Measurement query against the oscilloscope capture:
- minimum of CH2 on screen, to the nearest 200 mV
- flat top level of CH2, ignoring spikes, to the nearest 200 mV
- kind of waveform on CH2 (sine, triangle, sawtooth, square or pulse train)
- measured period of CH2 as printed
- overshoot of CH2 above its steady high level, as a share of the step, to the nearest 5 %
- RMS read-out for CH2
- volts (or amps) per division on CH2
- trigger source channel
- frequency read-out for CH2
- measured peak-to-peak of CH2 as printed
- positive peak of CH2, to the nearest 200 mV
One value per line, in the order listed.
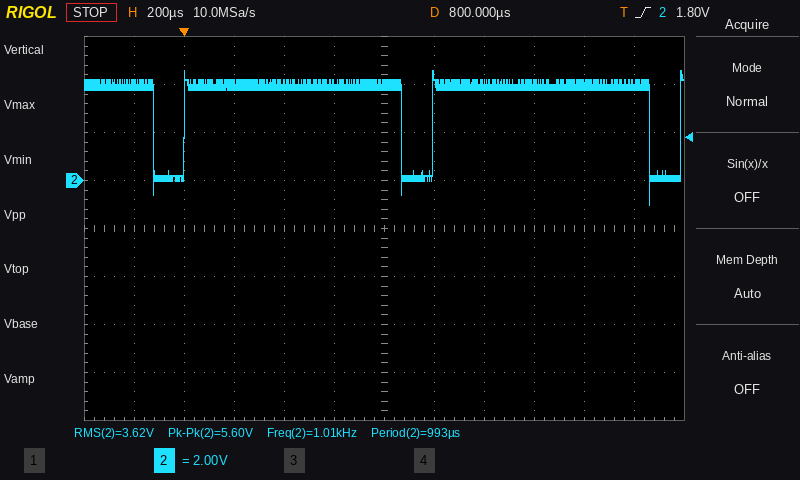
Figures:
-1.0 V
4.0 V
pulse train
993 µs
15 %
3.62 V
2 V
CH2
1.01 kHz
5.60 V
4.6 V
